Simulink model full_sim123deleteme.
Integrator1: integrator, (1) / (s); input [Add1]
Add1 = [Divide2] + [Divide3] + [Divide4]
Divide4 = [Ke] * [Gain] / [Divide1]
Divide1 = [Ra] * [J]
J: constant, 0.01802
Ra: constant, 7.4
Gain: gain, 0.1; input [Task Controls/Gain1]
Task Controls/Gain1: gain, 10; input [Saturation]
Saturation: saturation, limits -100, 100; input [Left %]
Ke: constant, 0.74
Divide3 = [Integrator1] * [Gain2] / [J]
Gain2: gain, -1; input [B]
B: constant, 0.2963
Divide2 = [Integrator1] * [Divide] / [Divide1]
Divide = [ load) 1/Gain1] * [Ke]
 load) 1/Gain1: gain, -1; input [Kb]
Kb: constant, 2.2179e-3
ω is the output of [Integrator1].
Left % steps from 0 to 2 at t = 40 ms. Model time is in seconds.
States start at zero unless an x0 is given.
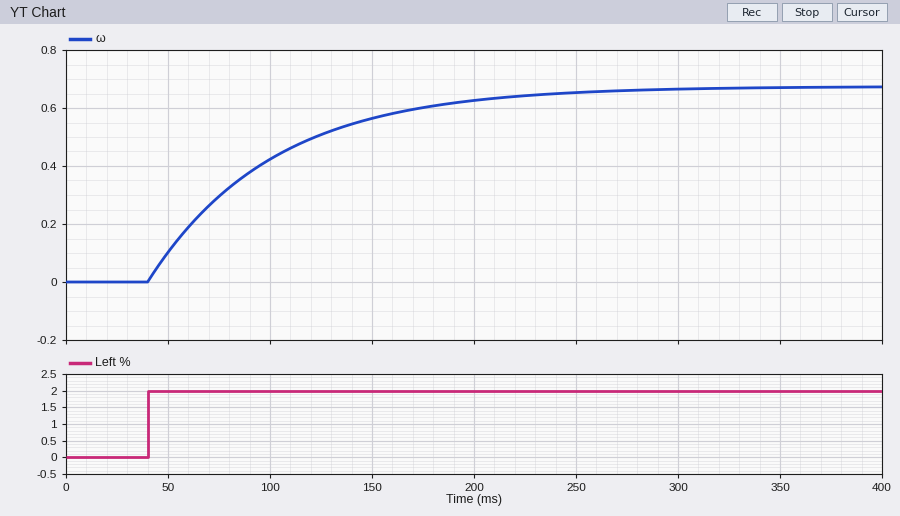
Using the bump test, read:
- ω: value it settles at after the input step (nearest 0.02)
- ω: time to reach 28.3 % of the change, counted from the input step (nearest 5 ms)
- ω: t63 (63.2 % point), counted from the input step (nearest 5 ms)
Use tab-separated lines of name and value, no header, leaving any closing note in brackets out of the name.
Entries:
ω: value it settles at after the input step	0.68
ω: time to reach 28.3 % of the change, counted from the input step	20 ms
ω: t63 (63.2 % point), counted from the input step	60 ms
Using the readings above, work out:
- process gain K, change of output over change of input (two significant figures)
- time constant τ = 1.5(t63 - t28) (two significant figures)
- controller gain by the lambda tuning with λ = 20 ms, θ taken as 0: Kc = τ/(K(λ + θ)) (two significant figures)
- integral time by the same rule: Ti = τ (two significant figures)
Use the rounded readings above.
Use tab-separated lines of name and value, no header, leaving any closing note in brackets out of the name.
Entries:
process gain K, change of output over change of input	0.34
time constant τ = 1.5(t63 - t28)	60 ms
controller gain by the lambda tuning with λ = 20 ms, θ taken as 0: Kc = τ/(K(λ + θ))	8.8
integral time by the same rule: Ti = τ	60 ms
